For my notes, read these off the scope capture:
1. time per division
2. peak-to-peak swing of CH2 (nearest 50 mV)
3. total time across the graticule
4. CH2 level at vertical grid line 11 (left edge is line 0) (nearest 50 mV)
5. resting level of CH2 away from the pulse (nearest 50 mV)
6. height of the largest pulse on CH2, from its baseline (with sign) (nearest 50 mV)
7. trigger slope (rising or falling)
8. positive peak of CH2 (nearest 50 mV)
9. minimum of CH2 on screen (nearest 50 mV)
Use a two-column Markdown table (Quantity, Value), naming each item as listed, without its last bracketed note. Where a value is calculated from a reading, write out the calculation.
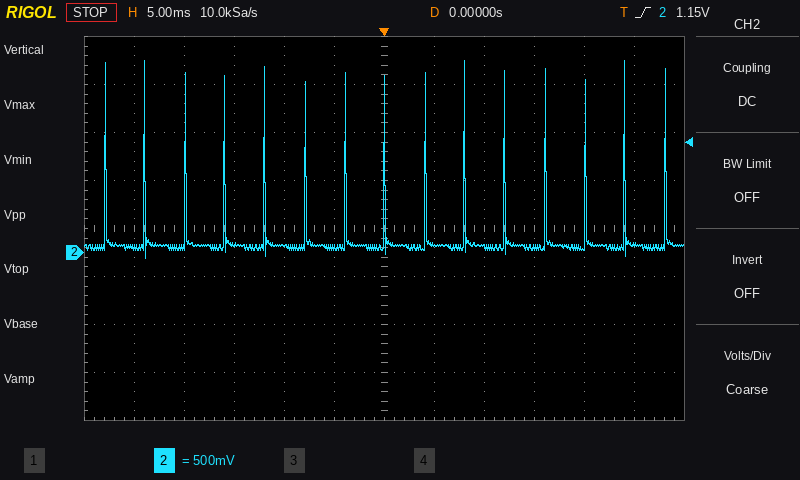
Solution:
| Quantity | Value |
|---|---|
| time per division | 5 ms |
| peak-to-peak swing of CH2 | 2.00 V − (-50 mV) = 2.05 V |
| total time across the graticule | 60 ms |
| CH2 level at vertical grid line 11 (left edge is line 0) | 100 mV |
| resting level of CH2 away from the pulse | 50 mV |
| height of the largest pulse on CH2, from its baseline (with sign) | 2.00 V − (50 mV) = +1.95 V |
| trigger slope | rising |
| positive peak of CH2 | 2.00 V |
| minimum of CH2 on screen | -50 mV |
